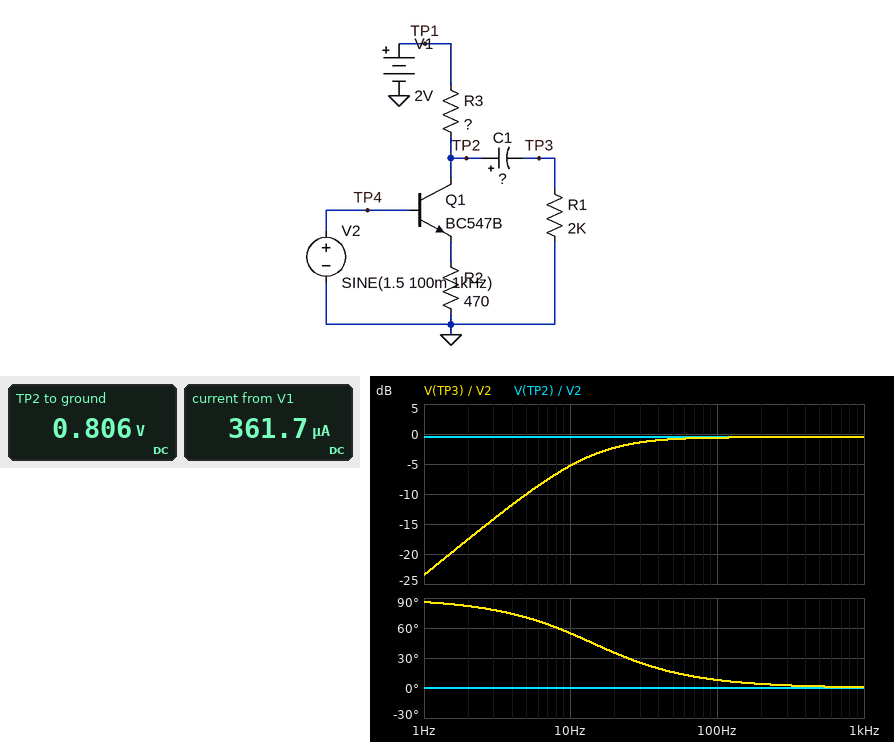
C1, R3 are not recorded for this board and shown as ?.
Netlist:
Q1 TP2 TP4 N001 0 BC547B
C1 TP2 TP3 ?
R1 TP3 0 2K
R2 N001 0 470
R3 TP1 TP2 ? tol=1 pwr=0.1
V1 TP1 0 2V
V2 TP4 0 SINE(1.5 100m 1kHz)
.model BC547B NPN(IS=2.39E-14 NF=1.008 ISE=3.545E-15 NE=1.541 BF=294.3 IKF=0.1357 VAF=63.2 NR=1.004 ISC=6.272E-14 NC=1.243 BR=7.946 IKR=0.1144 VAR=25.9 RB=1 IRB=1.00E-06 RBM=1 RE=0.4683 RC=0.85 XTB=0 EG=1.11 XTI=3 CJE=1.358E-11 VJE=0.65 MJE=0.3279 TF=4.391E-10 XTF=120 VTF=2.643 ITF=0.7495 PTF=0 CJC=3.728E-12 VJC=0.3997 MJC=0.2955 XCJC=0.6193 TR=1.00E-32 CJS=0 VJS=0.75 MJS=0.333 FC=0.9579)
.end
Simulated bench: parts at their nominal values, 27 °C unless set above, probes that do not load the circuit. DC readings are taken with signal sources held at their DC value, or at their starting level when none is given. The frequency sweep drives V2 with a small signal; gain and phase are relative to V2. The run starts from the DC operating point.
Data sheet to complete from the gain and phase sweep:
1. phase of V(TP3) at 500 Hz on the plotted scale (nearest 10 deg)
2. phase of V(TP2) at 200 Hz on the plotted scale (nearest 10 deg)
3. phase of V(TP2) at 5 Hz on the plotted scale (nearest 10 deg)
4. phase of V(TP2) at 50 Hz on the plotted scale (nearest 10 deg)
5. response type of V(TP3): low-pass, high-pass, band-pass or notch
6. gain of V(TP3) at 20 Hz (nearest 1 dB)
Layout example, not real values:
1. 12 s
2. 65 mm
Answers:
1. 0 deg
2. 0 deg
3. 0 deg
4. 0 deg
5. high-pass
6. -2 dB
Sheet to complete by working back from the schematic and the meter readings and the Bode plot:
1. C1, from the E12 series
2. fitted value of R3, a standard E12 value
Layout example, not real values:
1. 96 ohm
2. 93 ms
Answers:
1. 5.6 µF
2. 3.3 kΩ
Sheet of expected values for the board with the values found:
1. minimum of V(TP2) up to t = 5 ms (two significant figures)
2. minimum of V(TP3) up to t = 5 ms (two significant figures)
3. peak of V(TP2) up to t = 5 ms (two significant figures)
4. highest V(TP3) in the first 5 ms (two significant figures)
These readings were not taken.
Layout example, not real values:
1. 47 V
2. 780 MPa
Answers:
1. 710 mV
2. -95 mV
3. 900 mV
4. 94 mV
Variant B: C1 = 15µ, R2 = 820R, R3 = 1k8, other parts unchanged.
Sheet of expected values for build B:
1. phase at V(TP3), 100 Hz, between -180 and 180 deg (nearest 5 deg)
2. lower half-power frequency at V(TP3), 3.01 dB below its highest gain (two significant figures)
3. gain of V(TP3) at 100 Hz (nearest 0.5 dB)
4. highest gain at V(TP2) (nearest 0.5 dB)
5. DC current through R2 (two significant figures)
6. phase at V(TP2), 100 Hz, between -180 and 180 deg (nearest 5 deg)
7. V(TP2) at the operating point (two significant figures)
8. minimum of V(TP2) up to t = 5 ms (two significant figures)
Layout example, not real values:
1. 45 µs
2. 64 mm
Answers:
1. 5 deg
2. 5.1 Hz
3. -1.5 dB
4. -1.0 dB
5. 1.0 mA
6. 0 deg
7. 840 mV
8. 760 mV
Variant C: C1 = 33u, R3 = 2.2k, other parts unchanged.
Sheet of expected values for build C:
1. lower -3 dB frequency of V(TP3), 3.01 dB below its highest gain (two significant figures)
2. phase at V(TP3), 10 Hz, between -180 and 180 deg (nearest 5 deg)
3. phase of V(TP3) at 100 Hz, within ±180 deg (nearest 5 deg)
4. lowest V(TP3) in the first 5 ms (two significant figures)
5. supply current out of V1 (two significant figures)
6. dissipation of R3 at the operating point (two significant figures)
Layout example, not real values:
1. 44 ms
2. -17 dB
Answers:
1. 2.4 Hz
2. 15 deg
3. 0 deg
4. -92 mV
5. 540 µA
6. 640 µW
